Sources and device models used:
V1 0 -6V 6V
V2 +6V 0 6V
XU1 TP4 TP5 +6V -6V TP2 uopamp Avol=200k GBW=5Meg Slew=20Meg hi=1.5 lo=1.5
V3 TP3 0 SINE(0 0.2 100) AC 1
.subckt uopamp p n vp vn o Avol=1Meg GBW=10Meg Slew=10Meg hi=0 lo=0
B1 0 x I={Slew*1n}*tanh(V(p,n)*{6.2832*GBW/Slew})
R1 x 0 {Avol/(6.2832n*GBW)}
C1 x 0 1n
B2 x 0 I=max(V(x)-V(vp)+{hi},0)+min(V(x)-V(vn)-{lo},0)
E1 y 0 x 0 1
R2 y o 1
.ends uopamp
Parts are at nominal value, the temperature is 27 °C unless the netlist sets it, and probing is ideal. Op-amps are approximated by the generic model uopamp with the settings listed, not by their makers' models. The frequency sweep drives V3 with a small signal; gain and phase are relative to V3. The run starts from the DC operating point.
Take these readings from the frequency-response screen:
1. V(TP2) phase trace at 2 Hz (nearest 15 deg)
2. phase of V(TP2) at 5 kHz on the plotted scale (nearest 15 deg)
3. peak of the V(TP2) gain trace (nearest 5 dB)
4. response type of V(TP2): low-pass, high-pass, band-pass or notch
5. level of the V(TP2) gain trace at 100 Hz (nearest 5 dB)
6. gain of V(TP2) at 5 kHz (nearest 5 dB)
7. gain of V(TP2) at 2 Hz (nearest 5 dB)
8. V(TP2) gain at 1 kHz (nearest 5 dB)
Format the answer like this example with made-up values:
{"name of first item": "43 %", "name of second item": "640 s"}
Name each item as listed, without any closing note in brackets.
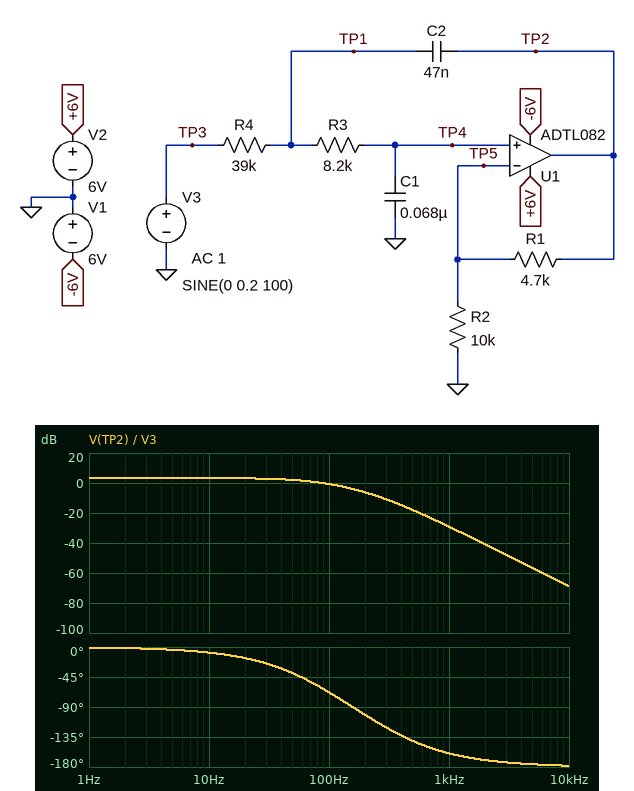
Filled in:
{"V(TP2) phase trace at 2 Hz": "0 deg", "phase of V(TP2) at 5 kHz on the plotted scale": "-180 deg", "peak of the V(TP2) gain trace": "5 dB", "response type of V(TP2): low-pass, high-pass, band-pass or notch": "low-pass", "level of the V(TP2) gain trace at 100 Hz": "0 dB", "gain of V(TP2) at 5 kHz": "-55 dB", "gain of V(TP2) at 2 Hz": "5 dB", "V(TP2) gain at 1 kHz": "-30 dB"}
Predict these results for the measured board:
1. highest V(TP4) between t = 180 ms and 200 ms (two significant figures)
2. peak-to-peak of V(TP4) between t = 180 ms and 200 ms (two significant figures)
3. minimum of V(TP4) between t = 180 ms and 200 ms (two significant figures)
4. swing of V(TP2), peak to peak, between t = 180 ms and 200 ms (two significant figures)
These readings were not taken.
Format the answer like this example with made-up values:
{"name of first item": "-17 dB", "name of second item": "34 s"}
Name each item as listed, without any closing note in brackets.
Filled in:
{"highest V(TP4) between t = 180 ms and 200 ms": "130 mV", "peak-to-peak of V(TP4) between t = 180 ms and 200 ms": "250 mV", "minimum of V(TP4) between t = 180 ms and 200 ms": "-130 mV", "swing of V(TP2), peak to peak, between t = 180 ms and 200 ms": "370 mV"}
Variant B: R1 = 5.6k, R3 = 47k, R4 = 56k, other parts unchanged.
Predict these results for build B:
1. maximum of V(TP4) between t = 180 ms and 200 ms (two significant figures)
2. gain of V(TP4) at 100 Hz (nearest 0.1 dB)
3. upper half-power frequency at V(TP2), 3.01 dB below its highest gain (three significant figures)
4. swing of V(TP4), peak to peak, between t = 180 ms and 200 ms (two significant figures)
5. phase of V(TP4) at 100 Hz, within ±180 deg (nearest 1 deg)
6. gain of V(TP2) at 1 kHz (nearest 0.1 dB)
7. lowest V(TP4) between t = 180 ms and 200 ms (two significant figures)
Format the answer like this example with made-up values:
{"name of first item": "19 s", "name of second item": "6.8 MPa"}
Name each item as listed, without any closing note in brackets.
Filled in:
{"maximum of V(TP4) between t = 180 ms and 200 ms": "48 mV", "gain of V(TP4) at 100 Hz": "-12.4 dB", "upper half-power frequency at V(TP2), 3.01 dB below its highest gain": "37.8 Hz", "swing of V(TP4), peak to peak, between t = 180 ms and 200 ms": "96 mV", "phase of V(TP4) at 100 Hz, within ±180 deg": "-124 deg", "gain of V(TP2) at 1 kHz": "-46.6 dB", "lowest V(TP4) between t = 180 ms and 200 ms": "-48 mV"}
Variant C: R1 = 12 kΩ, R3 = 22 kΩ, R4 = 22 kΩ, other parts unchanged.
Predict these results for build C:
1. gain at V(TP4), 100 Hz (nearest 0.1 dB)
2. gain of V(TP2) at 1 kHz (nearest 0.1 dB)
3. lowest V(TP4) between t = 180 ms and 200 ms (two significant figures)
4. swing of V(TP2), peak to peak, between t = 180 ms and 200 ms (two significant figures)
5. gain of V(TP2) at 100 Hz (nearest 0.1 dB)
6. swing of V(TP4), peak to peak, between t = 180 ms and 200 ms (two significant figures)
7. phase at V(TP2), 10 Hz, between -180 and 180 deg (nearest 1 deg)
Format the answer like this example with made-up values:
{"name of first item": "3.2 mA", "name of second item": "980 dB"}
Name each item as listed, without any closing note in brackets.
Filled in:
{"gain at V(TP4), 100 Hz": "-1.3 dB", "gain of V(TP2) at 1 kHz": "-28.9 dB", "lowest V(TP4) between t = 180 ms and 200 ms": "-170 mV", "swing of V(TP2), peak to peak, between t = 180 ms and 200 ms": "750 mV", "gain of V(TP2) at 100 Hz": "5.5 dB", "swing of V(TP4), peak to peak, between t = 180 ms and 200 ms": "340 mV", "phase at V(TP2), 10 Hz, between -180 and 180 deg": "-6 deg"}
